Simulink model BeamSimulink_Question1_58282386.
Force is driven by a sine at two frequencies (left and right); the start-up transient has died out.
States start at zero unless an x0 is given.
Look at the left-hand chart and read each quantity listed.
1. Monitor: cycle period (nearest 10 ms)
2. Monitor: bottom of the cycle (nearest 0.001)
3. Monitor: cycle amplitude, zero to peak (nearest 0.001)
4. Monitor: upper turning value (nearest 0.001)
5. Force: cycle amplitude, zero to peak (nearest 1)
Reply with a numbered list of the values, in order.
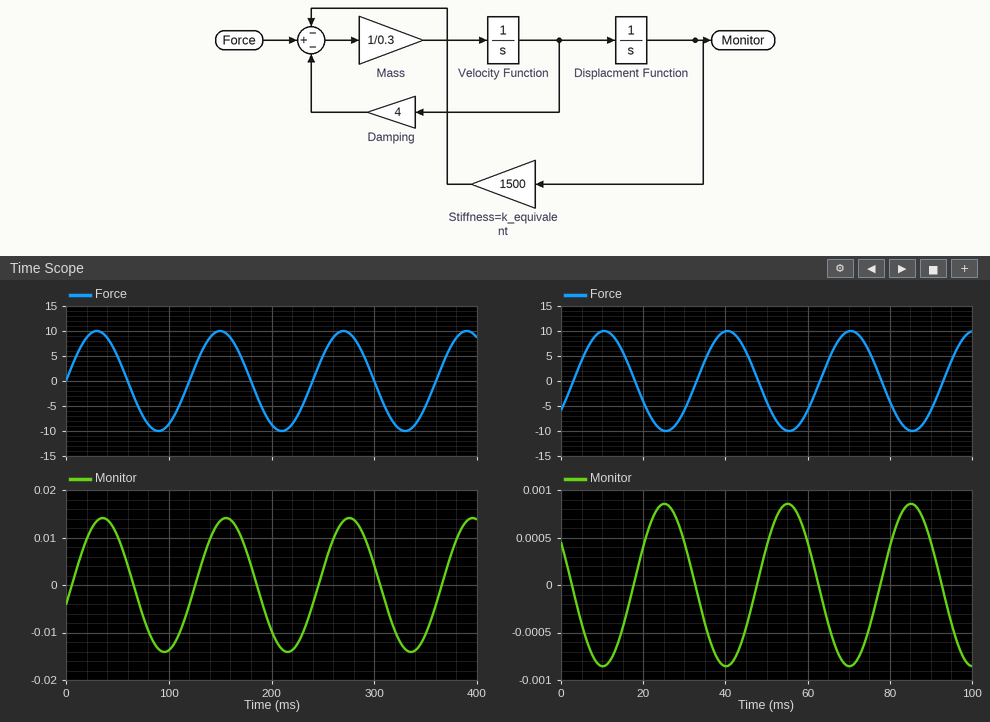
1. 120 ms
2. -0.014
3. 0.014
4. 0.014
5. 10
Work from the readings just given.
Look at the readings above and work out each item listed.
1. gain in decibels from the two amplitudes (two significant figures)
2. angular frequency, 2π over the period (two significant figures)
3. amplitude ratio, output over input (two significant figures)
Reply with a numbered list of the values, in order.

1. -57 dB
2. 0.052 rad/ms
3. 0.0014
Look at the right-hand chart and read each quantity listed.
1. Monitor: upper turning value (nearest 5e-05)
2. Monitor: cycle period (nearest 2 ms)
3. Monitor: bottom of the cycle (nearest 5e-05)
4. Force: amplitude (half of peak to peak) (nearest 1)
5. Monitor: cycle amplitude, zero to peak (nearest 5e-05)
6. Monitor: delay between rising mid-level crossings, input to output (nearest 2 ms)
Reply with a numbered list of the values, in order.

1. 0.00085
2. 30 ms
3. -0.00085
4. 10
5. 0.00085
6. 14 ms
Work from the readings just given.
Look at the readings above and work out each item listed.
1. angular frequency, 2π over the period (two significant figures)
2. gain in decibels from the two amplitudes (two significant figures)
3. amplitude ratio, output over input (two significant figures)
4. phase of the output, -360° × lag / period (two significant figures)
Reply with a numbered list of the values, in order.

1. 0.21 rad/ms
2. -81 dB
3. 0.000085
4. -170°
